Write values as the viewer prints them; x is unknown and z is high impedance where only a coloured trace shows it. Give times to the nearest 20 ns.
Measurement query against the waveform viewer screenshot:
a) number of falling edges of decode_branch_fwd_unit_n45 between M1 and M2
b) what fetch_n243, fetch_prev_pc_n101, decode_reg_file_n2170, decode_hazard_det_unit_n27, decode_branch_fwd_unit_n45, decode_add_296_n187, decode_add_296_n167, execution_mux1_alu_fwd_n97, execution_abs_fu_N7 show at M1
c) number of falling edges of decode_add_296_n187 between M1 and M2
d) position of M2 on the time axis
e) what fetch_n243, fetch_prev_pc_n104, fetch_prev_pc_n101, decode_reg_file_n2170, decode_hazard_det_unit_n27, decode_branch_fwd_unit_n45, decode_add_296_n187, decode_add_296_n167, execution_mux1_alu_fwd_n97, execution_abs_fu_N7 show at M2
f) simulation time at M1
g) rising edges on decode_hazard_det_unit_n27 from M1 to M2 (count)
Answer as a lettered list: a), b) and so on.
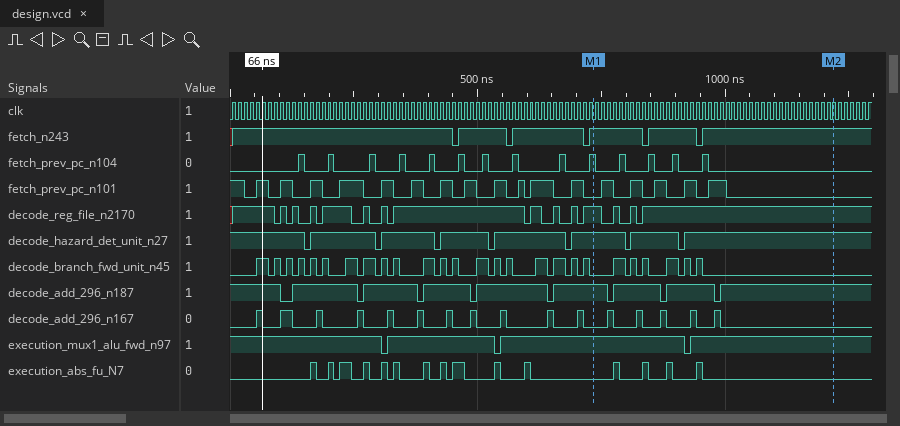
a) 6
b) fetch_n243=1, fetch_prev_pc_n101=0, decode_reg_file_n2170=1, decode_hazard_det_unit_n27=1, decode_branch_fwd_unit_n45=0, decode_add_296_n187=1, decode_add_296_n167=0, execution_mux1_alu_fwd_n97=1, execution_abs_fu_N7=0
c) 3
d) 1220 ns
e) fetch_n243=1, fetch_prev_pc_n104=0, fetch_prev_pc_n101=0, decode_reg_file_n2170=1, decode_hazard_det_unit_n27=1, decode_branch_fwd_unit_n45=0, decode_add_296_n187=1, decode_add_296_n167=0, execution_mux1_alu_fwd_n97=1, execution_abs_fu_N7=0
f) 740 ns
g) 2
